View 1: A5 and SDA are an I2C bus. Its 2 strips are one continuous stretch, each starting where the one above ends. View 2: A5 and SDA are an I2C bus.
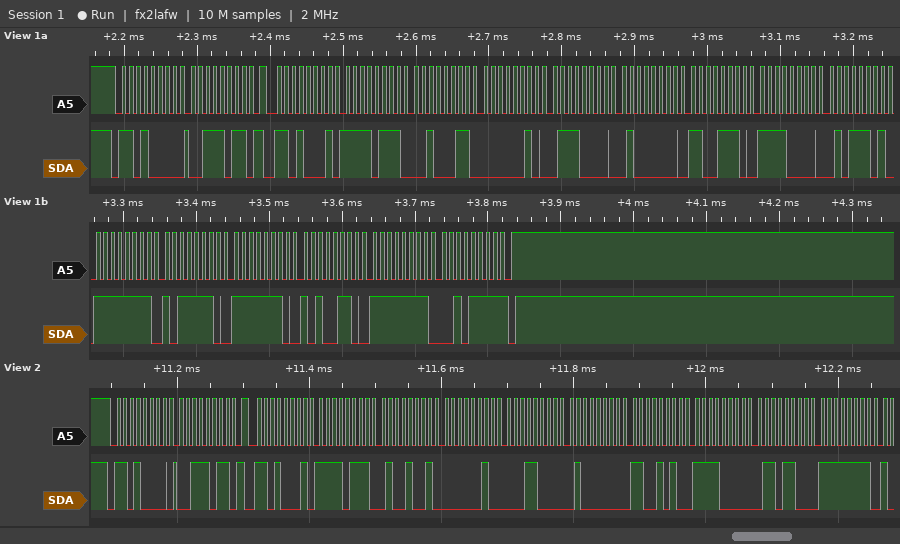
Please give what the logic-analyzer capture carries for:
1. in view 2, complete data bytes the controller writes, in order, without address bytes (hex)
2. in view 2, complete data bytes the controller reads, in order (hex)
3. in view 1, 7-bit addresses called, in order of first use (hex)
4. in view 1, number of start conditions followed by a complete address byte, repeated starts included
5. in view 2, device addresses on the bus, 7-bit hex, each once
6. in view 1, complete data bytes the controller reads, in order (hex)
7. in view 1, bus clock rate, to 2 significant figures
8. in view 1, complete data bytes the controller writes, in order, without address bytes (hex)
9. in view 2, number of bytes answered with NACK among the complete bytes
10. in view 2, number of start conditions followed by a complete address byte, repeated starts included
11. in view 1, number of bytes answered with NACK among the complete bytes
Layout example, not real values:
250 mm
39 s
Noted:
3B
F7 49 02 18 40 CA F0 6C FF
0x68
2
0x68
F7 23 02 70 40 CE F0 5D FF BE FE A6 FF 2F
100 kHz
3B
0
2
1
